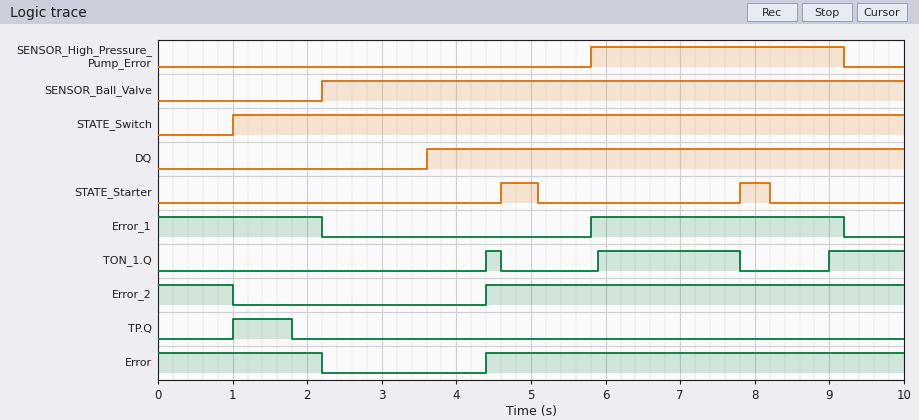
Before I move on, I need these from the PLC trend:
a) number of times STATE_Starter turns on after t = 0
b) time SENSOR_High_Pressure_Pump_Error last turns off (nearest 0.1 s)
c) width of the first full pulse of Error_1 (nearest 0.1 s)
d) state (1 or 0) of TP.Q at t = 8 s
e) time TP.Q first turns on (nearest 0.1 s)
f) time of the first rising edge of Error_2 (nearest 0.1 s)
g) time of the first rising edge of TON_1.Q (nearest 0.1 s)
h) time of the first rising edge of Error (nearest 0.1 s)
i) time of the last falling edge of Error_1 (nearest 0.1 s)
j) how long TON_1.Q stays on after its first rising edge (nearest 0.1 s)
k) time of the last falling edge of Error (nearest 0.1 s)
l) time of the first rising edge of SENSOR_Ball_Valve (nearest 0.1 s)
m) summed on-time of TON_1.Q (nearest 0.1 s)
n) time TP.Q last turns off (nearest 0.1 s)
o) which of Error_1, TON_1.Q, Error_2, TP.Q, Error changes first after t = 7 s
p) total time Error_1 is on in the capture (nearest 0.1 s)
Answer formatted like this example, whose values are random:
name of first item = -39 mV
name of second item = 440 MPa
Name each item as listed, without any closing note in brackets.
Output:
number of times STATE_Starter turns on after t = 0 = 2
time SENSOR_High_Pressure_Pump_Error last turns off = 9.2 s
width of the first full pulse of Error_1 = 3.4 s
state (1 or 0) of TP.Q at t = 8 s = 0
time TP.Q first turns on = 1.0 s
time of the first rising edge of Error_2 = 4.4 s
time of the first rising edge of TON_1.Q = 4.4 s
time of the first rising edge of Error = 4.4 s
time of the last falling edge of Error_1 = 9.2 s
how long TON_1.Q stays on after its first rising edge = 0.2 s
time of the last falling edge of Error = 2.2 s
time of the first rising edge of SENSOR_Ball_Valve = 2.2 s
summed on-time of TON_1.Q = 3.1 s
time TP.Q last turns off = 1.8 s
which of Error_1, TON_1.Q, Error_2, TP.Q, Error changes first after t = 7 s = TON_1.Q
total time Error_1 is on in the capture = 5.6 s
